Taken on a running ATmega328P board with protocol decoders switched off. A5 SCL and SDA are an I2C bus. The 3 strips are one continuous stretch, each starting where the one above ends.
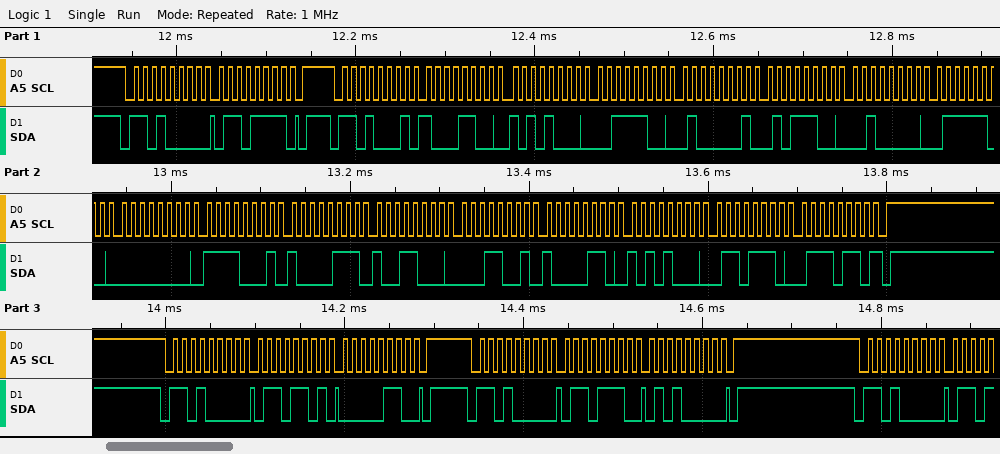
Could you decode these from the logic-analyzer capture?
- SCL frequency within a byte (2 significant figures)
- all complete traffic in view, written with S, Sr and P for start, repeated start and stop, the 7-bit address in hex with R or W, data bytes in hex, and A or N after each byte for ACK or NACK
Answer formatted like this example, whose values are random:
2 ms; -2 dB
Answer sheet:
100 kHz; S 68W A 6F A P S 68R A 8C A A8 A 3C A 41 A 5C A 20 A 7C A 00 A F1 A 87 A 98 A 19 A 86 A A8 A 6E A 76 N P S 68W A 6D A 06 A P S 68W A 6E A 50 A P S 68W A
